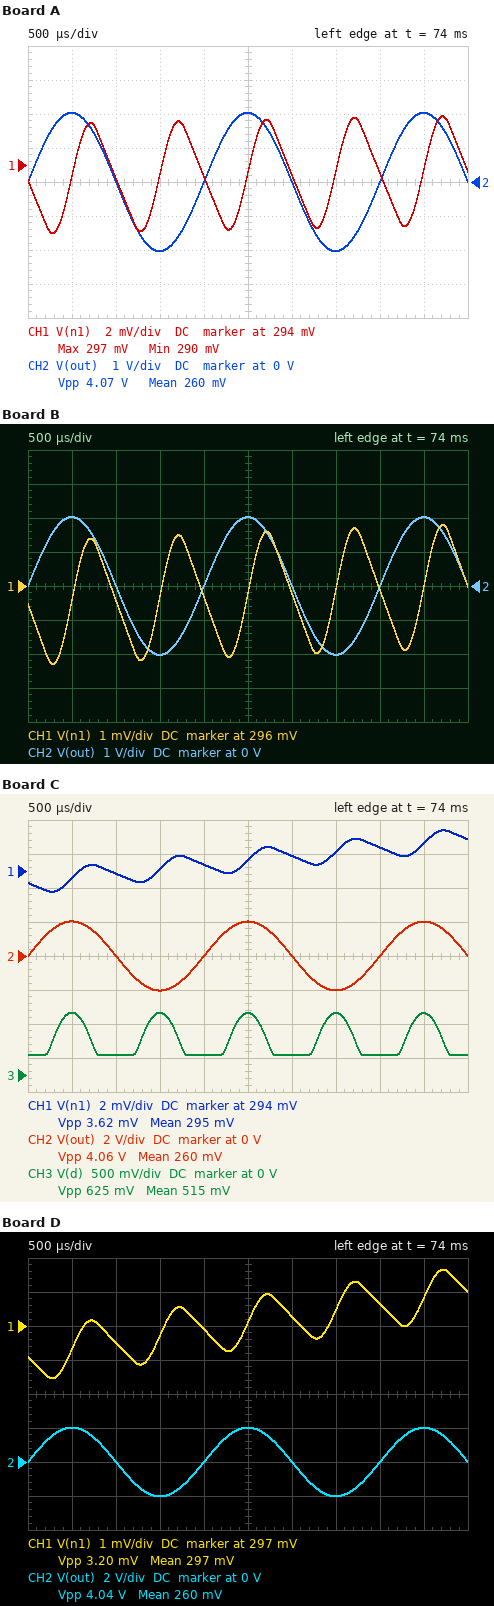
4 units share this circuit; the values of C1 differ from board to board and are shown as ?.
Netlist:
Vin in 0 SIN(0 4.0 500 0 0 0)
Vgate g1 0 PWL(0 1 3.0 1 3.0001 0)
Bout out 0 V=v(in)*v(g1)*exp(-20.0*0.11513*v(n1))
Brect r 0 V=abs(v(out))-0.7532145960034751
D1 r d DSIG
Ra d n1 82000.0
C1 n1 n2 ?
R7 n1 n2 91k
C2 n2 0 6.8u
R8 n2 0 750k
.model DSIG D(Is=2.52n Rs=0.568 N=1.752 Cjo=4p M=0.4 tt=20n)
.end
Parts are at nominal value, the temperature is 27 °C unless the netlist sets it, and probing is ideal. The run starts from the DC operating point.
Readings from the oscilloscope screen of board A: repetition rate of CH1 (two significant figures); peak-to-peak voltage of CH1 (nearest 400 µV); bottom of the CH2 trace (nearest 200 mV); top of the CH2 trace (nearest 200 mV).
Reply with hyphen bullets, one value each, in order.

- 1.0 kHz
- 6.8 mV
- -2.0 V
- 2.0 V
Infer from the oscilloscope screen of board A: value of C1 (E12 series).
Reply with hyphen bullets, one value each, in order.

- 220 nF
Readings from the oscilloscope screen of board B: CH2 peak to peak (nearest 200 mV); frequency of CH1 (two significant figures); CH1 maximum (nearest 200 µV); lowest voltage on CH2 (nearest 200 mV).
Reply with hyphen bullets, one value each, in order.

- 4.0 V
- 1.0 kHz
- 297.8 mV
- -2.0 V
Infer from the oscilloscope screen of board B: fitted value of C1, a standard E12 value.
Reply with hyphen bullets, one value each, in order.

- 390 nF
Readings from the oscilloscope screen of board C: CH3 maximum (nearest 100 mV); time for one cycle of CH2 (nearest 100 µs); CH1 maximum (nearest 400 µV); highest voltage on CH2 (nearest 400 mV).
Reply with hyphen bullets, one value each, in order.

- 900 mV
- 2.0 ms
- 296.4 mV
- 2.0 V
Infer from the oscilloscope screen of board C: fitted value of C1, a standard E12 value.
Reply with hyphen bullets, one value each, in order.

- 1.2 µF
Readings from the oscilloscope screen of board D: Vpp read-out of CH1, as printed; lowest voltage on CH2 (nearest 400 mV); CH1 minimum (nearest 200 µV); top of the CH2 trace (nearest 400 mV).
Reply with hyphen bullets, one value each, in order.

- 3.20 mV
- -2.0 V
- 295.4 mV
- 2.0 V
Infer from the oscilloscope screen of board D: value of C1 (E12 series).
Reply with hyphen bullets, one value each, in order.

- 1 µF
